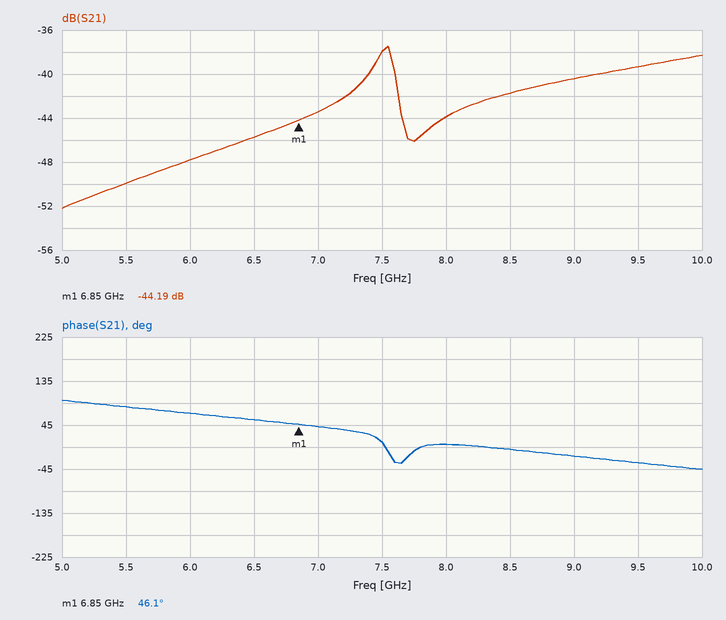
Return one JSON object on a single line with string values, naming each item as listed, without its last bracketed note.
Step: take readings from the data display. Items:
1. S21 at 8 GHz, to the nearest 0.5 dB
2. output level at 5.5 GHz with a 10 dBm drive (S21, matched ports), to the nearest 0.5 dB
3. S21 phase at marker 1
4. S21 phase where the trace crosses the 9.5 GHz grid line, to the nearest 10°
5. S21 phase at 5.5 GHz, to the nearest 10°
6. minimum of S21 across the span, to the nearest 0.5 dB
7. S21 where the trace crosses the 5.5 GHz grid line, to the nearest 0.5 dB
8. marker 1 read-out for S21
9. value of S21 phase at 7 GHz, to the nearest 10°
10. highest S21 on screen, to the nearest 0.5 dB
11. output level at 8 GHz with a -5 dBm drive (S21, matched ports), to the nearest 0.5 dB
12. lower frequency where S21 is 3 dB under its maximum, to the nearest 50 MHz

{"S21 at 8 GHz, to the nearest 0.5 dB": "-44.0 dB", "output level at 5.5 GHz with a 10 dBm drive (S21, matched ports), to the nearest 0.5 dB": "-40.0 dBm", "S21 phase at marker 1": "46.1°", "S21 phase where the trace crosses the 9.5 GHz grid line, to the nearest 10°": "-30°", "S21 phase at 5.5 GHz, to the nearest 10°": "80°", "minimum of S21 across the span, to the nearest 0.5 dB": "-52.0 dB", "S21 where the trace crosses the 5.5 GHz grid line, to the nearest 0.5 dB": "-50.0 dB", "marker 1 read-out for S21": "-44.19 dB", "value of S21 phase at 7 GHz, to the nearest 10°": "40°", "highest S21 on screen, to the nearest 0.5 dB": "-37.5 dB", "output level at 8 GHz with a -5 dBm drive (S21, matched ports), to the nearest 0.5 dB": "-49.0 dBm", "lower frequency where S21 is 3 dB under its maximum, to the nearest 50 MHz": "7.35 GHz"}
